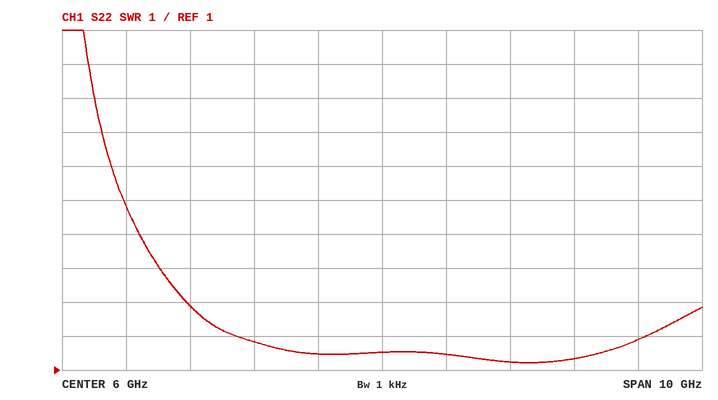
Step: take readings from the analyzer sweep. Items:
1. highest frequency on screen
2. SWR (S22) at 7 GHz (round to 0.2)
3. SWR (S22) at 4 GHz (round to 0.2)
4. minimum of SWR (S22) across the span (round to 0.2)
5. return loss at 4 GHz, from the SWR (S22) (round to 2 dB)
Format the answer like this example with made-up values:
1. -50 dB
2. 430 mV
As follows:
1. 11 GHz
2. 1.4
3. 1.8
4. 1.2
5. 10 dB
